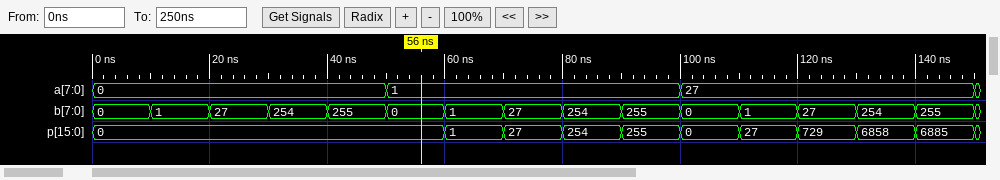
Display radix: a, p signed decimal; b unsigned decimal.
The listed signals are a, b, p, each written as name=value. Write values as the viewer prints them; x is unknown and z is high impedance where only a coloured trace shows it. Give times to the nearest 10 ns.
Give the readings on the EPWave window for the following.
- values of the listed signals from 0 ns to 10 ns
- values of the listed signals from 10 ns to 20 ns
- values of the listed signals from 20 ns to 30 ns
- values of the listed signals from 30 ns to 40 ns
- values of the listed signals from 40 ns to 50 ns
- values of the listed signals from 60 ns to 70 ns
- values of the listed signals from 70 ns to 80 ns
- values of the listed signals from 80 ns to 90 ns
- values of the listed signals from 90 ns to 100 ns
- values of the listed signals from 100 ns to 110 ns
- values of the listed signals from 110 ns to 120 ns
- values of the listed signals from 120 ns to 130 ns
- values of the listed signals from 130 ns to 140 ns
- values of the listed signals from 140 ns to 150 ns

a=0, b=0, p=0
a=0, b=1, p=0
a=0, b=27, p=0
a=0, b=254, p=0
a=0, b=255, p=0
a=1, b=1, p=1
a=1, b=27, p=27
a=1, b=254, p=254
a=1, b=255, p=255
a=27, b=0, p=0
a=27, b=1, p=27
a=27, b=27, p=729
a=27, b=254, p=6858
a=27, b=255, p=6885
